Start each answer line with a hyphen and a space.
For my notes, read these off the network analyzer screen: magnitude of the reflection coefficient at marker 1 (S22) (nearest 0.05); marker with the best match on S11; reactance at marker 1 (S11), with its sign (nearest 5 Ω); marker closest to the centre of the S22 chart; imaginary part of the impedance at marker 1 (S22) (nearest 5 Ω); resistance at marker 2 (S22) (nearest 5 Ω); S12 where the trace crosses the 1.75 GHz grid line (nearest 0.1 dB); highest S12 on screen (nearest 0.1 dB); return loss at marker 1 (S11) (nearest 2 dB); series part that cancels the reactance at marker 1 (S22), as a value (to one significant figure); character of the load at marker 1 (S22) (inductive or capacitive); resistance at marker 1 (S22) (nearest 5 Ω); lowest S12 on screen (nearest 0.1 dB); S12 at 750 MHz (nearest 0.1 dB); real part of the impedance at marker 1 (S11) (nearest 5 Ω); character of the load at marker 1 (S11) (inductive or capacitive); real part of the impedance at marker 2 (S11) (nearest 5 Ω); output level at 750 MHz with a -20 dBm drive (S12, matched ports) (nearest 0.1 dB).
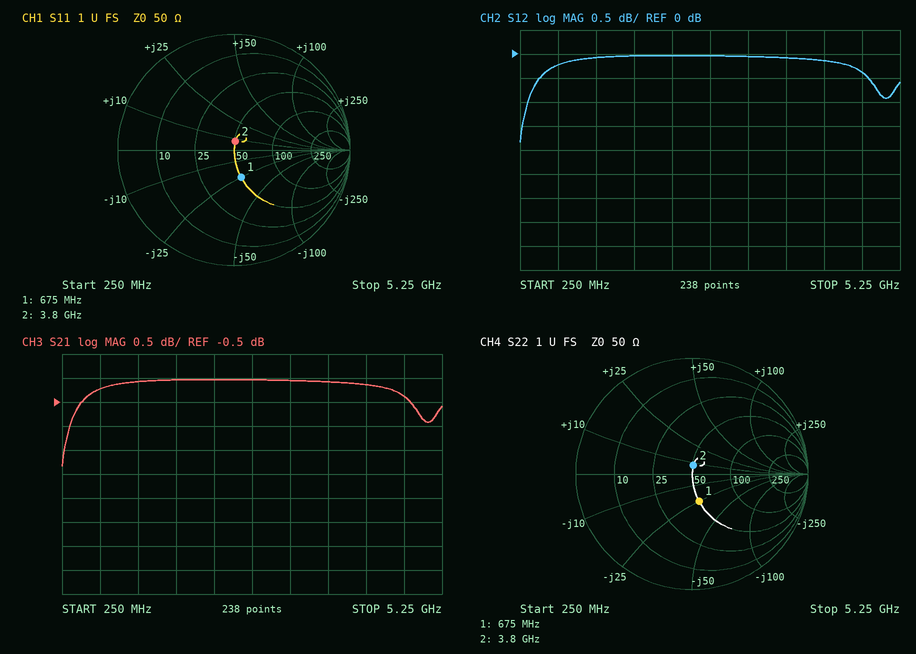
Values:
- 0.25
- marker 2
- -25 Ω
- marker 2
- -25 Ω
- 50 Ω
- 0.0 dB
- 0.0 dB
- 12 dB
- 6 nH
- capacitive
- 50 Ω
- -1.8 dB
- -0.2 dB
- 50 Ω
- capacitive
- 50 Ω
- -20.2 dBm
